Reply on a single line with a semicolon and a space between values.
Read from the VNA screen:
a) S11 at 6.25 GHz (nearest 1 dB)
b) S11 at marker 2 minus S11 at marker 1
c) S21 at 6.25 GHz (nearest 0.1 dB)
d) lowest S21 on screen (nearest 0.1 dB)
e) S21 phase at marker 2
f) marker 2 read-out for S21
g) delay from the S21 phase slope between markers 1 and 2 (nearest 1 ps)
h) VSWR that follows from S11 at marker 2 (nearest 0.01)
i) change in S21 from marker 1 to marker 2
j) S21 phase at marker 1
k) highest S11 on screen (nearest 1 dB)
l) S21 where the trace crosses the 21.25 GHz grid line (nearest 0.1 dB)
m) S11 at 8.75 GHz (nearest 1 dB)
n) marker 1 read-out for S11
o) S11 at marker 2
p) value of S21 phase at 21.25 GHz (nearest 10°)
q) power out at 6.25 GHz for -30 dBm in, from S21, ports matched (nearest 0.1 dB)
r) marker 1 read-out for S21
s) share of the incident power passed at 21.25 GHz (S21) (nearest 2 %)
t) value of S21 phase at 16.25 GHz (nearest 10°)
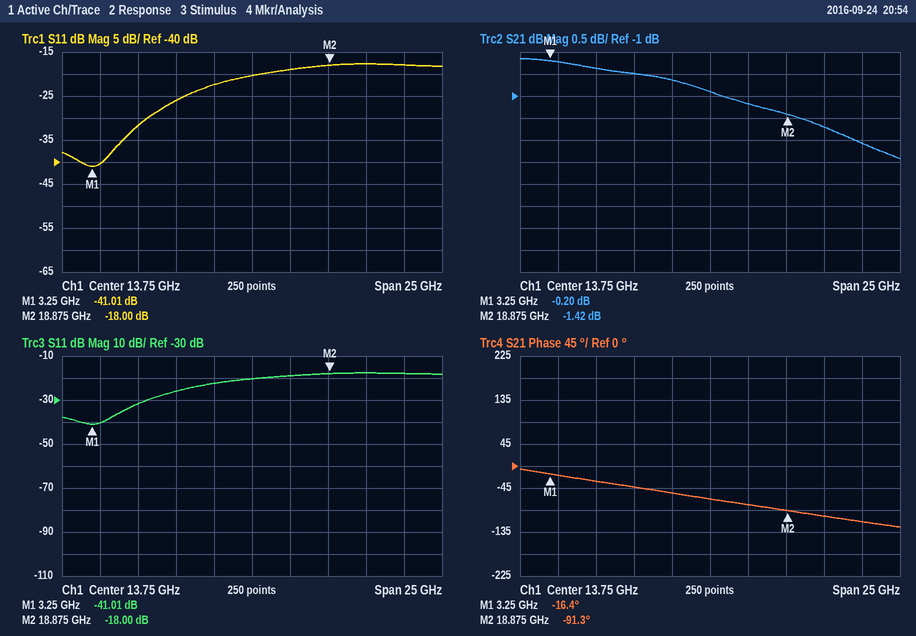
-32 dB; 23.01 dB; -0.4 dB; -2.4 dB; -91.3°; -1.42 dB; 13 ps; 1.29; -1.22 dB; -16.4°; -18 dB; -1.7 dB; -26 dB; -41.01 dB; -18.00 dB; -100°; -30.4 dBm; -0.20 dB; 68 %; -80°
